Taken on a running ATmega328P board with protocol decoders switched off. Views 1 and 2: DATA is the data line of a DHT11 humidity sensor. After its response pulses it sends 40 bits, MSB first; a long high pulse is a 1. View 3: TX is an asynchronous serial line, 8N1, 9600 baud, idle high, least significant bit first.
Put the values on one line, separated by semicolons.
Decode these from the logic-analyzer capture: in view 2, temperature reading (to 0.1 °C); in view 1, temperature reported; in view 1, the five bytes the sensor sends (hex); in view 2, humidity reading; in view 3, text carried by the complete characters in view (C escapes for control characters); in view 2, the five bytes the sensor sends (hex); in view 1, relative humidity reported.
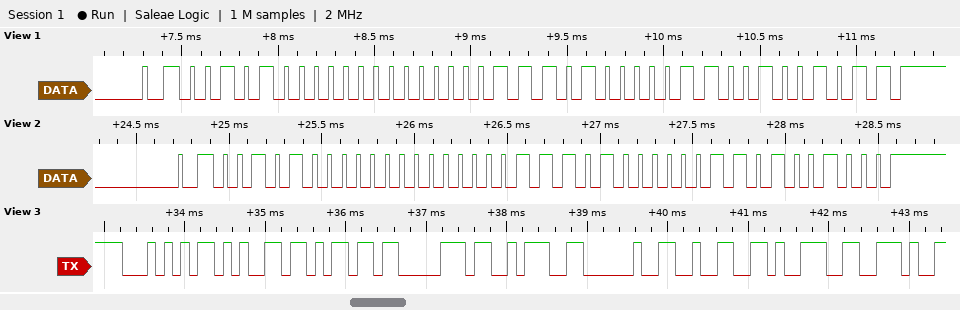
29.3 °C; 29.6 °C; 28 00 1D 06 4B; 40 %; "Temp: 29."; 28 00 1D 03 48; 40 %
